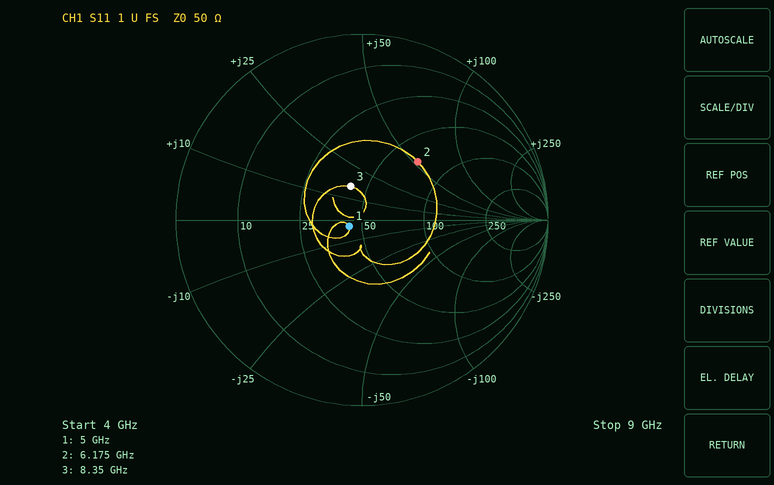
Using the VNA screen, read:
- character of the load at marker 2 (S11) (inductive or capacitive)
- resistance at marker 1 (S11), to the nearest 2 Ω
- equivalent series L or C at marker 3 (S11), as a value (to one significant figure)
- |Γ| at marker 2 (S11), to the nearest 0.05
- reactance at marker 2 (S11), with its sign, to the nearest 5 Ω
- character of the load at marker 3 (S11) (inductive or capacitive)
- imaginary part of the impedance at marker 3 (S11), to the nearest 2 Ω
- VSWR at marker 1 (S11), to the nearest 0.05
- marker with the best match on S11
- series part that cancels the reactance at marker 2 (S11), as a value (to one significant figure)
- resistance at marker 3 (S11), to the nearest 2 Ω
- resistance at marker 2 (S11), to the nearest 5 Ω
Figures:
inductive
44 Ω
300 pH
0.45
+55 Ω
inductive
+16 Ω
1.15
marker 1
500 fF
42 Ω
70 Ω
